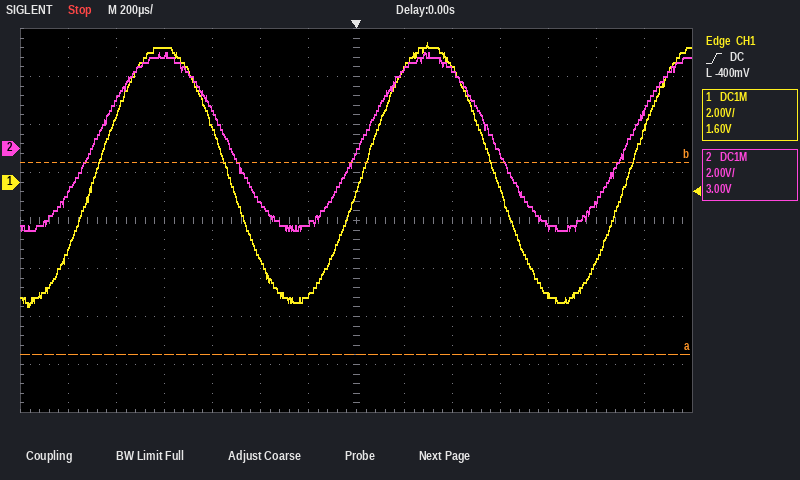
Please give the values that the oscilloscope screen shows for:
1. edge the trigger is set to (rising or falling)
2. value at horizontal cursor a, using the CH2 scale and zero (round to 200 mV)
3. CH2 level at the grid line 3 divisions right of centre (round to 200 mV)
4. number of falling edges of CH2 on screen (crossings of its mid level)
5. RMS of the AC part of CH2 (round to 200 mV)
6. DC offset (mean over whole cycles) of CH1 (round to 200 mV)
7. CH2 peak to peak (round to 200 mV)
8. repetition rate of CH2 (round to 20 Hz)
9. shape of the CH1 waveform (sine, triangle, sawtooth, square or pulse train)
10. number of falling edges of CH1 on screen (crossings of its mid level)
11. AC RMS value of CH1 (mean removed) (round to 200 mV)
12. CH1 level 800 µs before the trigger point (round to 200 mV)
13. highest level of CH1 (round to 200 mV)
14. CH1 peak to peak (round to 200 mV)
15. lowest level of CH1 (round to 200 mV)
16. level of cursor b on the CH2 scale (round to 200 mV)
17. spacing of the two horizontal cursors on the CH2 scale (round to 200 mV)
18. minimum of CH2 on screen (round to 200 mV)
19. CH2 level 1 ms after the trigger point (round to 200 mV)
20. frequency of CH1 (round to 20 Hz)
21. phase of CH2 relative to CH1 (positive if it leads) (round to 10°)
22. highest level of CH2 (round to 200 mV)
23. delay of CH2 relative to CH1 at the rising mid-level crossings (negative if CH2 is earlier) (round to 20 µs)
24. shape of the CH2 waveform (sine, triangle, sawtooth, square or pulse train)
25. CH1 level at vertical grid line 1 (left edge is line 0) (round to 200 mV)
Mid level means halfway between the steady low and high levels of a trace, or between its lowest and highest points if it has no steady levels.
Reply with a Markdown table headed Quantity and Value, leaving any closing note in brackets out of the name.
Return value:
| Quantity | Value |
|---|---|
| edge the trigger is set to | rising |
| value at horizontal cursor a, using the CH2 scale and zero | -8.6 V |
| CH2 level at the grid line 3 divisions right of centre | -200 mV |
| number of falling edges of CH2 on screen | 2 |
| RMS of the AC part of CH2 | 2.6 V |
| DC offset (mean over whole cycles) of CH1 | 400 mV |
| CH2 peak to peak | 7.4 V |
| repetition rate of CH2 | 900 Hz |
| shape of the CH1 waveform | sine |
| number of falling edges of CH1 on screen | 2 |
| AC RMS value of CH1 (mean removed) | 3.8 V |
| CH1 level 800 µs before the trigger point | 5.6 V |
| highest level of CH1 | 5.8 V |
| CH1 peak to peak | 11.0 V |
| lowest level of CH1 | -5.2 V |
| level of cursor b on the CH2 scale | -600 mV |
| spacing of the two horizontal cursors on the CH2 scale | 8.0 V |
| minimum of CH2 on screen | -3.4 V |
| CH2 level 1 ms after the trigger point | -2.2 V |
| frequency of CH1 | 900 Hz |
| phase of CH2 relative to CH1 (positive if it leads) | 0° |
| highest level of CH2 | 4.0 V |
| delay of CH2 relative to CH1 at the rising mid-level crossings (negative if CH2 is earlier) | 0 µs |
| shape of the CH2 waveform | sine |
| CH1 level at vertical grid line 1 (left edge is line 0) | -2.8 V |
